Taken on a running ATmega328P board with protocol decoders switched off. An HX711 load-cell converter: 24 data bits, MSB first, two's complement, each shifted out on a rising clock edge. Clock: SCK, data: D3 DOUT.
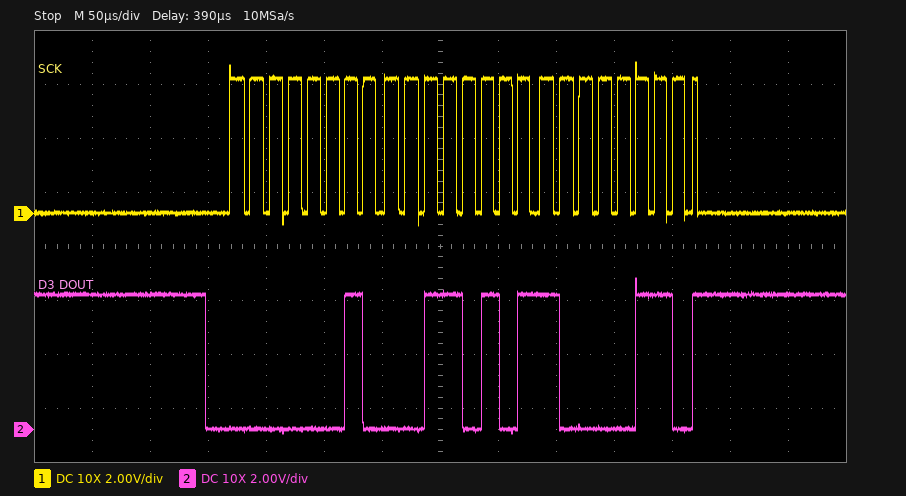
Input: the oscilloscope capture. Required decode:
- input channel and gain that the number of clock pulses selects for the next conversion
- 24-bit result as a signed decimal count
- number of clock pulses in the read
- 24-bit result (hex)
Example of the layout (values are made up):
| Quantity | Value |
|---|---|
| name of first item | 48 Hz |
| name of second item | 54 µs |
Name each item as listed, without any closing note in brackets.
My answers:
| Quantity | Value |
|---|---|
| input channel and gain that the number of clock pulses selects for the next conversion | channel A, gain 128 |
| 24-bit result as a signed decimal count | 144774 |
| number of clock pulses in the read | 25 |
| 24-bit result | 0x023586 |
